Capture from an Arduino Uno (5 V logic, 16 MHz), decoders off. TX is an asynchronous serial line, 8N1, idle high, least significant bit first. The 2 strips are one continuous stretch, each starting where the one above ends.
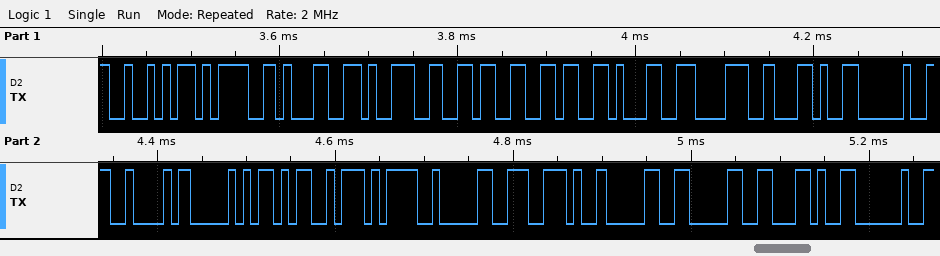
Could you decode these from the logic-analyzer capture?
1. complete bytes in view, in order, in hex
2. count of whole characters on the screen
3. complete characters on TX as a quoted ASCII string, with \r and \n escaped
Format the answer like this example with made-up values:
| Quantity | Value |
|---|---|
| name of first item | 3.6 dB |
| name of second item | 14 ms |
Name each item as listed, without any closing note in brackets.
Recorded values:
| Quantity | Value |
|---|---|
| complete bytes in view, in order, in hex | 52 3D 31 39 36 36 31 38 2C 20 42 50 4D 3D 30 2E 30 30 2C 20 |
| count of whole characters on the screen | 20 |
| complete characters on TX as a quoted ASCII string, with \r and \n escaped | "R=196618, BPM=0.00, " |
